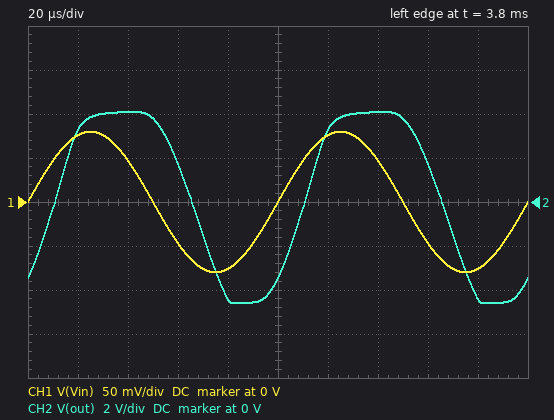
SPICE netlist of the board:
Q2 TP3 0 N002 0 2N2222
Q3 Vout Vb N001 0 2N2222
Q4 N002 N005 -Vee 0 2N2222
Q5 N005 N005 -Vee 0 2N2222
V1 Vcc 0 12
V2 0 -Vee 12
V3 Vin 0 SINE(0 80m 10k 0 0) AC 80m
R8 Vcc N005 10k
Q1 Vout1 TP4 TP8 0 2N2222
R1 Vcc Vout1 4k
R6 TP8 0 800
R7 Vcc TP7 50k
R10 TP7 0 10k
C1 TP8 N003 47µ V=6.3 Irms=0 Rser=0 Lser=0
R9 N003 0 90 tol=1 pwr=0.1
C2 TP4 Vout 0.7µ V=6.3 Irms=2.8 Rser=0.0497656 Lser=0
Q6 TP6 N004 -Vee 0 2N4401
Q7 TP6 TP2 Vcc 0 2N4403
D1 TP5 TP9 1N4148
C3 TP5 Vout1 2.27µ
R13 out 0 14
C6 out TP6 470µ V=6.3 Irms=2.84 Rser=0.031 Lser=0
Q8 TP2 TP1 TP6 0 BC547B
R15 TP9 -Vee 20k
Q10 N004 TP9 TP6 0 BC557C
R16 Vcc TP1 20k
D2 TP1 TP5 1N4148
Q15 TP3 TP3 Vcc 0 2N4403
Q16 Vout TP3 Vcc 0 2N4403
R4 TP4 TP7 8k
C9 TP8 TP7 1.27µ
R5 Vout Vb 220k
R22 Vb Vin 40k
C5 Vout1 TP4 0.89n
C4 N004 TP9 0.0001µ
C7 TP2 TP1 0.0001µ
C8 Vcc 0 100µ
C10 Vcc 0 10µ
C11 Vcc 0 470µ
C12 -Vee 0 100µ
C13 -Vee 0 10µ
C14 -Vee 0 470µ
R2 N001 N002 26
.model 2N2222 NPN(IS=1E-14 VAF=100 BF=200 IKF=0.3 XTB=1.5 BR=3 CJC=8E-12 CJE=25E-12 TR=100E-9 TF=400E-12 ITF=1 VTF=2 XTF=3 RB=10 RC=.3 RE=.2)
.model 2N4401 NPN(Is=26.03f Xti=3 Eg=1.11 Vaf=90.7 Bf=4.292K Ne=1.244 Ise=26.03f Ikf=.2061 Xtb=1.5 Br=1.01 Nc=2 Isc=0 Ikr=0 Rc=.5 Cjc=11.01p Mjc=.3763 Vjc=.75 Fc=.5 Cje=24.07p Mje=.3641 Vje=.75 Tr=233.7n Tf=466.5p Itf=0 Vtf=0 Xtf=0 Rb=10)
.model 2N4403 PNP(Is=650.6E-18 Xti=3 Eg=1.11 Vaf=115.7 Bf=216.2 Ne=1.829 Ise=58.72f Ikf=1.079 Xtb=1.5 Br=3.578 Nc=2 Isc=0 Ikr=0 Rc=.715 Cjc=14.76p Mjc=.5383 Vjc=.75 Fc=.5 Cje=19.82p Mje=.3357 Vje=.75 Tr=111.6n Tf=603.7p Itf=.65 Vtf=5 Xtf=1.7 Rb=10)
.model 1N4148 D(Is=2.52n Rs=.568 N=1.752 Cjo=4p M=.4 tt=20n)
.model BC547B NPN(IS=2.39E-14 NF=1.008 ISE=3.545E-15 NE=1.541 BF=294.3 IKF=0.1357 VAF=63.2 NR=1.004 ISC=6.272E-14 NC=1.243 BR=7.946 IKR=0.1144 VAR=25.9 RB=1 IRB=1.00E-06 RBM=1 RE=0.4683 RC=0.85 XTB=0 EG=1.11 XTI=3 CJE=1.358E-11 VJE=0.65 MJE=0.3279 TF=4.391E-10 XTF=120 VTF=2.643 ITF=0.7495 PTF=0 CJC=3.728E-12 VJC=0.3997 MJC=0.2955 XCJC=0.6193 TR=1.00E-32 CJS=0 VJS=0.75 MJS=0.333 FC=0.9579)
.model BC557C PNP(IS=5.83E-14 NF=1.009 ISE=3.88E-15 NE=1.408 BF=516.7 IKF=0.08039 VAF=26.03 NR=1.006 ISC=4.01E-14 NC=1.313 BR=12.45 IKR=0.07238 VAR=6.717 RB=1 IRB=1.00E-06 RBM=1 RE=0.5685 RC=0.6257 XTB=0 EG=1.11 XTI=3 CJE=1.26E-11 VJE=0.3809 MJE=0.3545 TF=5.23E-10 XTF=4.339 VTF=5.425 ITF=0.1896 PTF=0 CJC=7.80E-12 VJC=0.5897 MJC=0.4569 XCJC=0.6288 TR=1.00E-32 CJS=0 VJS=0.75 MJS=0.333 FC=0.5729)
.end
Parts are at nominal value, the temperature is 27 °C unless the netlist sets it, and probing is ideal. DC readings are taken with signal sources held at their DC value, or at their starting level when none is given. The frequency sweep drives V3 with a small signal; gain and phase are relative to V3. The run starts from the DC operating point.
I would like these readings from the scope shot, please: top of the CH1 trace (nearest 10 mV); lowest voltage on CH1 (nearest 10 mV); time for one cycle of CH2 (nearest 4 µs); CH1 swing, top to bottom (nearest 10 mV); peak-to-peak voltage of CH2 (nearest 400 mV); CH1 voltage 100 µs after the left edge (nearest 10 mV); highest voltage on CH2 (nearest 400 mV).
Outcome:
80 mV
-80 mV
100 µs
160 mV
8.8 V
0 V
4.0 V
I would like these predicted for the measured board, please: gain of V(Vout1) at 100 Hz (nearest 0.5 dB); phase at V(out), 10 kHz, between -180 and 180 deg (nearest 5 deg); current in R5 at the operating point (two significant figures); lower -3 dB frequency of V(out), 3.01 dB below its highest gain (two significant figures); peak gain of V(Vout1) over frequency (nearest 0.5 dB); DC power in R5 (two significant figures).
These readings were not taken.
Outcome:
42.5 dB
-55 deg
7.4 µA
46 Hz
43.0 dB
12 µW
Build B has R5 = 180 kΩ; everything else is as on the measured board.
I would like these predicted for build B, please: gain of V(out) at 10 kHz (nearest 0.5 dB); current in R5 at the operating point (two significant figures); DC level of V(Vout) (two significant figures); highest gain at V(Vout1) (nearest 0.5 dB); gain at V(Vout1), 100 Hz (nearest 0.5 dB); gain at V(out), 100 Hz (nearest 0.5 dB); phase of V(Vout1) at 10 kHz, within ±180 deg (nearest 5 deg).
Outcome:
37.5 dB
7.5 µA
1.4 V
41.5 dB
41.0 dB
40.0 dB
-50 deg
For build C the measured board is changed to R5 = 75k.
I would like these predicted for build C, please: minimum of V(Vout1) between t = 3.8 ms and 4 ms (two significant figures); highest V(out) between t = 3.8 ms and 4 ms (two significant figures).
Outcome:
2.4 V
3.1 V
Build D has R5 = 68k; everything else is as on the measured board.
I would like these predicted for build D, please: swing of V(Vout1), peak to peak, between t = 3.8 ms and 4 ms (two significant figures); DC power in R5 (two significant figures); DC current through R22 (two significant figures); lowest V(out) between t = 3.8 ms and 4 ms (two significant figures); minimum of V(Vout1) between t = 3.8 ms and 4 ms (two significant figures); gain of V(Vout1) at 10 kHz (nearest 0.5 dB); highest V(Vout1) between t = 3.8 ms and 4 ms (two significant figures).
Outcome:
6.2 V
3.9 µW
970 nA
-3.1 V
2.7 V
32.0 dB
8.9 V
